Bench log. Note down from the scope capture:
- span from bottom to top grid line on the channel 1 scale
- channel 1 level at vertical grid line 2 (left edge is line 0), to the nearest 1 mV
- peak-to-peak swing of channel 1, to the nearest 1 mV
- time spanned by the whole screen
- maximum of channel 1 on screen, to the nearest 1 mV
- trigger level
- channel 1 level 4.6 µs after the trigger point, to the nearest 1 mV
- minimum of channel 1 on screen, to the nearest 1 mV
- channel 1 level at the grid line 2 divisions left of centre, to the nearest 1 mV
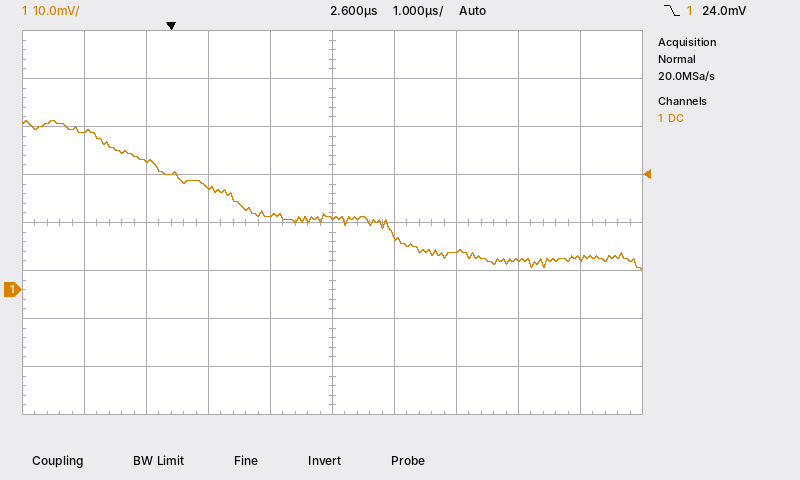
80 mV
27 mV
31 mV
10 µs
35 mV
24.0 mV
8 mV
4 mV
21 mV
